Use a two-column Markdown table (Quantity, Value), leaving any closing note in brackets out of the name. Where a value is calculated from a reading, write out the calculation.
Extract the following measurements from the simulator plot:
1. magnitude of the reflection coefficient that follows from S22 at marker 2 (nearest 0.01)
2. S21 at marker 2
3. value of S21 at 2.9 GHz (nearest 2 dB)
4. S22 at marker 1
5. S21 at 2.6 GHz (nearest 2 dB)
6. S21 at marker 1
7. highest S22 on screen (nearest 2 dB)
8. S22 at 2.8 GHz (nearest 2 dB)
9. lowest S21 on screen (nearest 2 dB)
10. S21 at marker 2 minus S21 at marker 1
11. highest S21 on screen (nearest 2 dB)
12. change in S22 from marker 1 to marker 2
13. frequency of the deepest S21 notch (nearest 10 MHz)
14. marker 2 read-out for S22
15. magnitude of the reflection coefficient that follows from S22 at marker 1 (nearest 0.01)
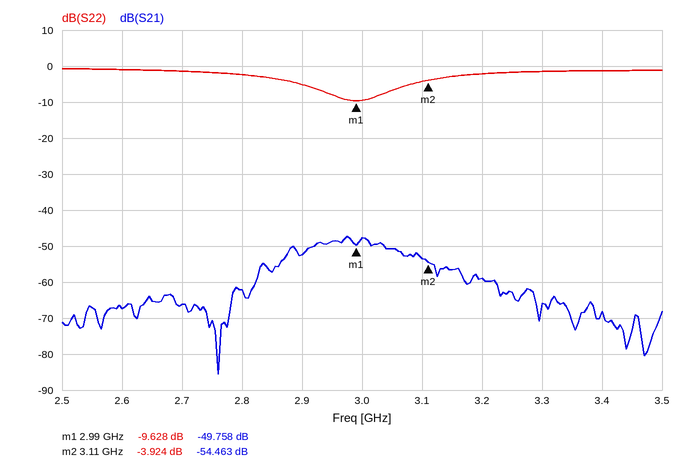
| Quantity | Value |
|---|---|
| magnitude of the reflection coefficient that follows from S22 at marker 2 | 10^(-3.924/20) ≈ 0.64 |
| S21 at marker 2 | -54.463 dB |
| value of S21 at 2.9 GHz | -52 dB |
| S22 at marker 1 | -9.628 dB |
| S21 at 2.6 GHz | -68 dB |
| S21 at marker 1 | -49.758 dB |
| highest S22 on screen | 0 dB |
| S22 at 2.8 GHz | -2 dB |
| lowest S21 on screen | -86 dB |
| S21 at marker 2 minus S21 at marker 1 | -54.463 − (-49.758) = -4.705 dB |
| highest S21 on screen | -48 dB |
| change in S22 from marker 1 to marker 2 | -3.924 − (-9.628) = 5.704 dB |
| frequency of the deepest S21 notch | 2.76 GHz |
| marker 2 read-out for S22 | -3.924 dB |
| magnitude of the reflection coefficient that follows from S22 at marker 1 | 10^(-9.628/20) ≈ 0.33 |
